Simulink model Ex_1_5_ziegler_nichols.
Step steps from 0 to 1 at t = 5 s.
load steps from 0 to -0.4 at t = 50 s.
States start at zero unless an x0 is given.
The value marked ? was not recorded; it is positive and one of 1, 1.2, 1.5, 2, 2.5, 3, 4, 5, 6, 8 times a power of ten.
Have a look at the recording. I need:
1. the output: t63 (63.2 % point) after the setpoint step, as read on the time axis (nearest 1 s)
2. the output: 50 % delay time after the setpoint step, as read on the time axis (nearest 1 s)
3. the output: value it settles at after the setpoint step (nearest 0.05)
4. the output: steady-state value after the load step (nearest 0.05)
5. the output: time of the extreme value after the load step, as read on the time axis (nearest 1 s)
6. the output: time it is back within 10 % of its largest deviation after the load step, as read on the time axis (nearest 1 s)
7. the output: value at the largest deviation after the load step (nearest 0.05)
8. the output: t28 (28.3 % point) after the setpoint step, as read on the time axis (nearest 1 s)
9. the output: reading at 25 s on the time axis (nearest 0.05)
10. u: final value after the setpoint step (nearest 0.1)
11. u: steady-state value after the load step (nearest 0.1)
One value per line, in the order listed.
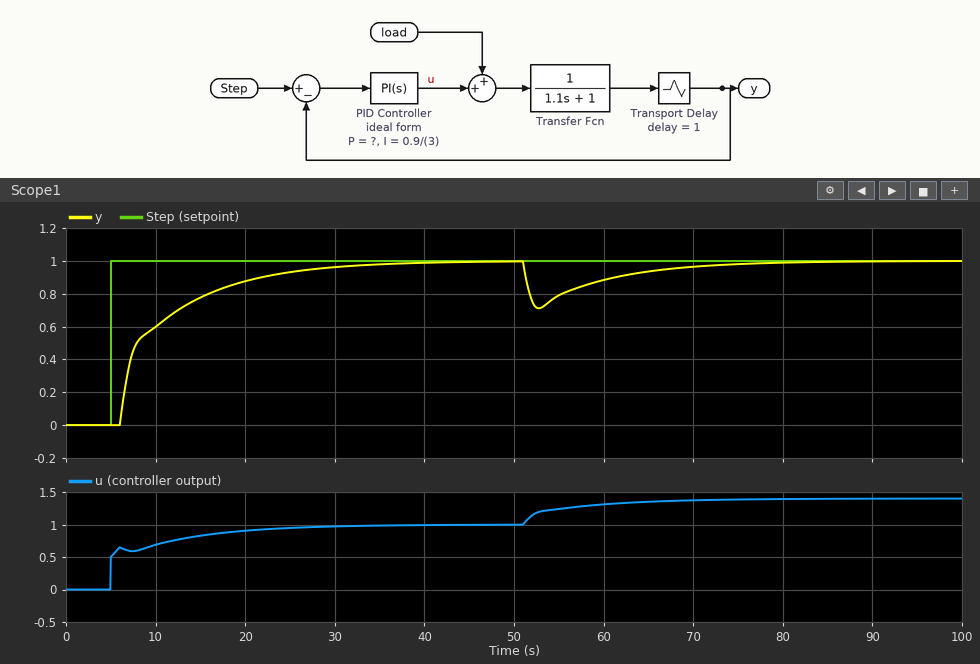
11 s
8 s
1.00
1.00
53 s
72 s
0.70
7 s
0.95
1.0
1.4
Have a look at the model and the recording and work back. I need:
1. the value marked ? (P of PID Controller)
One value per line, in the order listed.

0.5
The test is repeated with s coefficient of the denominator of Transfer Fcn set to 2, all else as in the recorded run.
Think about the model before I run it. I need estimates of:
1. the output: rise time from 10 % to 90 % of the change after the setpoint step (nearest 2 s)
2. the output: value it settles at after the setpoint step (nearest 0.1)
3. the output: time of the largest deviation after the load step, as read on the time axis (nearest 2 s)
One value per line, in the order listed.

14 s
1.0
54 s
